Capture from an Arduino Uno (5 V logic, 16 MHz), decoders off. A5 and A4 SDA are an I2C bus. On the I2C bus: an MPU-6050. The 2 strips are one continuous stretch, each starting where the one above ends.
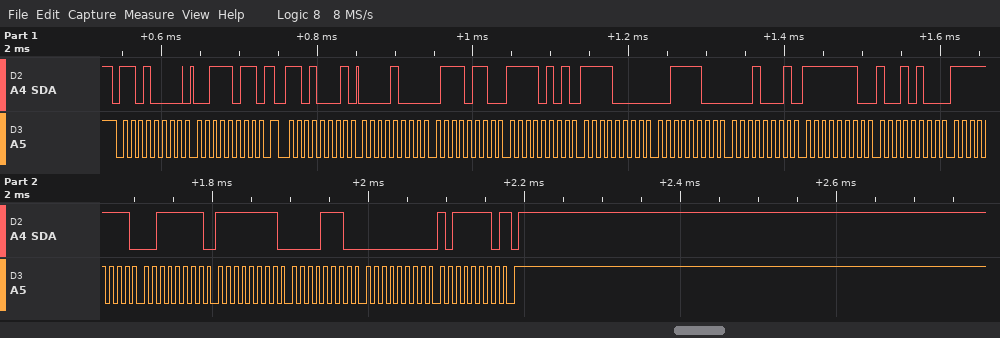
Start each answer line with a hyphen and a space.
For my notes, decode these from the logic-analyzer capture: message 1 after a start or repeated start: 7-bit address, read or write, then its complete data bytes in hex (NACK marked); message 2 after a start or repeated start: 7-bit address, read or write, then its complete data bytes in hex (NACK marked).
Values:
- 0x68 write: 3B
- 0x68 read: 08 76 F5 F0 3C 11 FE 94 FF 3F FF 0E 00 BE NACK
